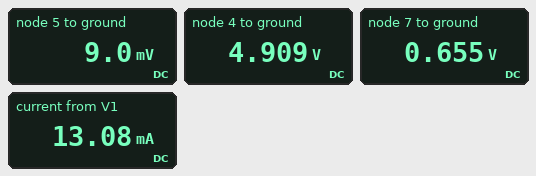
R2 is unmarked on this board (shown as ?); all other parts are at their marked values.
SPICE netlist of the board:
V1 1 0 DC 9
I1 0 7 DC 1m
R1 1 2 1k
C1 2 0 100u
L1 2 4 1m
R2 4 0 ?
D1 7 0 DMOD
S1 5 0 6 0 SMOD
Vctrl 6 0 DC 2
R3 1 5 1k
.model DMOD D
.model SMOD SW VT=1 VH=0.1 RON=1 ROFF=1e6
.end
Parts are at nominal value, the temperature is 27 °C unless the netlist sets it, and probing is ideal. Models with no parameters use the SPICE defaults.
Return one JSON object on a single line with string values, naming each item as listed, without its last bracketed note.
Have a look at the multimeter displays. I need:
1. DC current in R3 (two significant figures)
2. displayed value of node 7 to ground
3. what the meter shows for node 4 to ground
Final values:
{"DC current in R3": "9.0 mA", "displayed value of node 7 to ground": "0.655 V", "what the meter shows for node 4 to ground": "4.909 V"}
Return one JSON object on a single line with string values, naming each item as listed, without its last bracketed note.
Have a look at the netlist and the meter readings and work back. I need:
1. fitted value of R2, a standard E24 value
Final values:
{"fitted value of R2, a standard E24 value": "1.2 kΩ"}
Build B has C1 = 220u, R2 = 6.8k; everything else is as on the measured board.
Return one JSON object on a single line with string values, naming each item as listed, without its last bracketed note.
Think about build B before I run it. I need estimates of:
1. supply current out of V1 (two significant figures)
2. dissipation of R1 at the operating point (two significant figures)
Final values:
{"supply current out of V1": "10 mA", "dissipation of R1 at the operating point": "1.3 mW"}
